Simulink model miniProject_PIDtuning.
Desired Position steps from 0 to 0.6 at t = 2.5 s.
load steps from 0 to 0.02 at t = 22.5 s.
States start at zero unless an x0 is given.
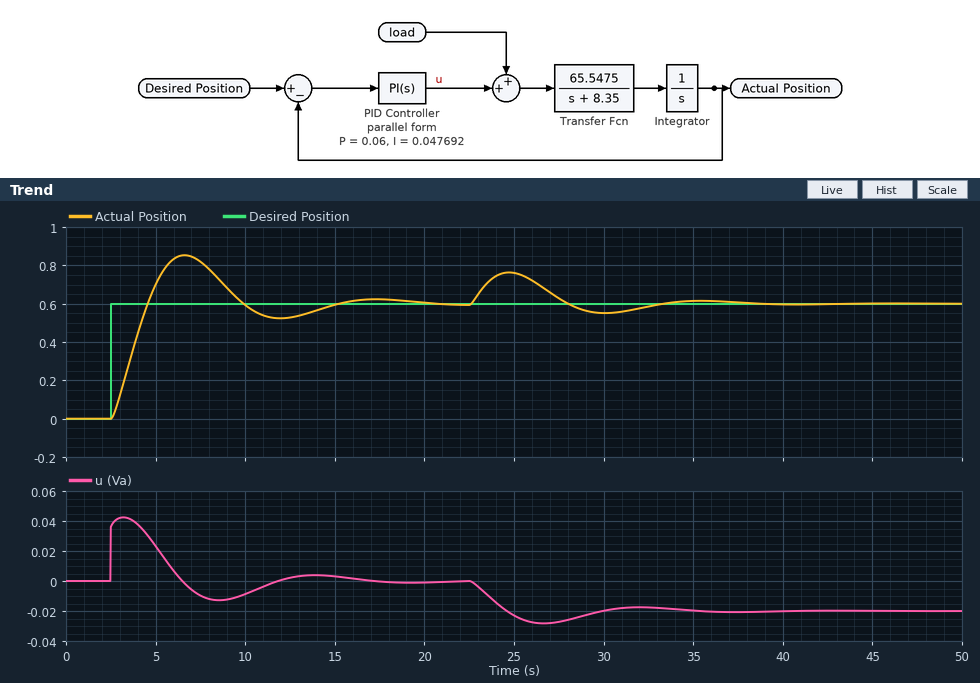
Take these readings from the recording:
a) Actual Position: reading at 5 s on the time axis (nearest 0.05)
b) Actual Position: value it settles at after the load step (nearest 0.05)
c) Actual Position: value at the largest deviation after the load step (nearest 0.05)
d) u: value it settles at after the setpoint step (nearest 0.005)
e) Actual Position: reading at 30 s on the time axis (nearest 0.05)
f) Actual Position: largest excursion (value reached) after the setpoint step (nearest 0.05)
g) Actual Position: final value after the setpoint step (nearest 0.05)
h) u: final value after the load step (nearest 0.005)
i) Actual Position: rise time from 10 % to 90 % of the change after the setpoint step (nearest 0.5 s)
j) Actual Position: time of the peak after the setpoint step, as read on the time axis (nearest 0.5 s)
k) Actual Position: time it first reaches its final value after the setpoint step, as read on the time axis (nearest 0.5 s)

0.70
0.60
0.75
0.000
0.55
0.85
0.60
-0.020
1.5 s
6.5 s
4.5 s
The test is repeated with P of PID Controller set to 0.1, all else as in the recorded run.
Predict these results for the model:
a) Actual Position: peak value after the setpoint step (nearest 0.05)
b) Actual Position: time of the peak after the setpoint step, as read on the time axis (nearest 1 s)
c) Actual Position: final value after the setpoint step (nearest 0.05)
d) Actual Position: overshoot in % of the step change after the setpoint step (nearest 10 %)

0.75
6 s
0.60
30 %
